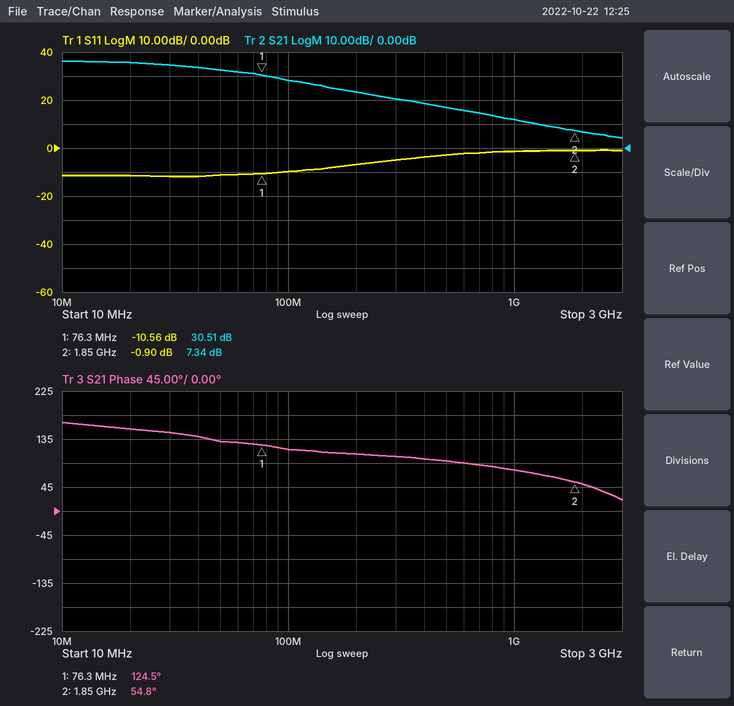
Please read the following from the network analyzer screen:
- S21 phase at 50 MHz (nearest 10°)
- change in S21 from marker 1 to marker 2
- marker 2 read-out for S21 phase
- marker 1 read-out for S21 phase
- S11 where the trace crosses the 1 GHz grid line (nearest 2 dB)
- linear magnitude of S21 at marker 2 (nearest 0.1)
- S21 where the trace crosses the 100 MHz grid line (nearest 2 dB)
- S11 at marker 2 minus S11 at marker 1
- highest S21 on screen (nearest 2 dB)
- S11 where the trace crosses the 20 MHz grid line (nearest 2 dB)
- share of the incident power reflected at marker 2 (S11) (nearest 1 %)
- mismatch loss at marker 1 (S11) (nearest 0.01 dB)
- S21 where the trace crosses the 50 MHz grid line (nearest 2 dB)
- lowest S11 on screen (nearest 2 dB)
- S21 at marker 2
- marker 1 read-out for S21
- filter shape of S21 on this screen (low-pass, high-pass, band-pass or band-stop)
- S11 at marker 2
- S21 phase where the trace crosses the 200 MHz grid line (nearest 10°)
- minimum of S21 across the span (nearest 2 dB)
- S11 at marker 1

130°
-23.17 dB
54.8°
124.5°
-2 dB
2.3
28 dB
9.66 dB
36 dB
-12 dB
81 %
0.40 dB
32 dB
-12 dB
7.34 dB
30.51 dB
low-pass
-0.90 dB
110°
4 dB
-10.56 dB
